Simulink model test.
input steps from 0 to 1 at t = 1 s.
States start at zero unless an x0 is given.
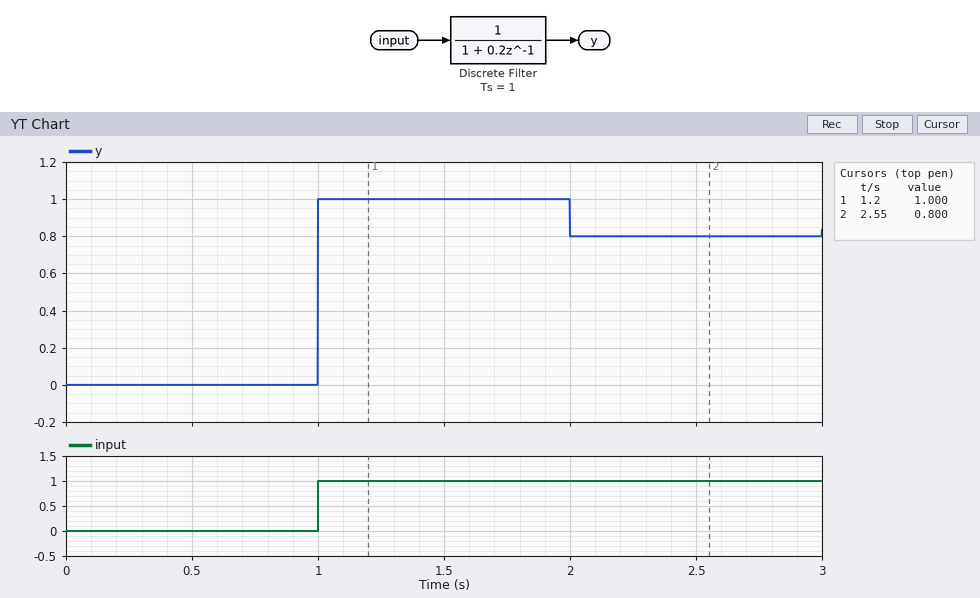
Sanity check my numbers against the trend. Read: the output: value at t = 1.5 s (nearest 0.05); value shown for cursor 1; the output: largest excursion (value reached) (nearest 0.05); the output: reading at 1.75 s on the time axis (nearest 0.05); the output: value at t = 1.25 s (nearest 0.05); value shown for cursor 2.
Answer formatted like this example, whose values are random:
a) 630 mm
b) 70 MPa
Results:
a) 1.00
b) 1.000
c) 1.00
d) 1.00
e) 1.00
f) 0.800
